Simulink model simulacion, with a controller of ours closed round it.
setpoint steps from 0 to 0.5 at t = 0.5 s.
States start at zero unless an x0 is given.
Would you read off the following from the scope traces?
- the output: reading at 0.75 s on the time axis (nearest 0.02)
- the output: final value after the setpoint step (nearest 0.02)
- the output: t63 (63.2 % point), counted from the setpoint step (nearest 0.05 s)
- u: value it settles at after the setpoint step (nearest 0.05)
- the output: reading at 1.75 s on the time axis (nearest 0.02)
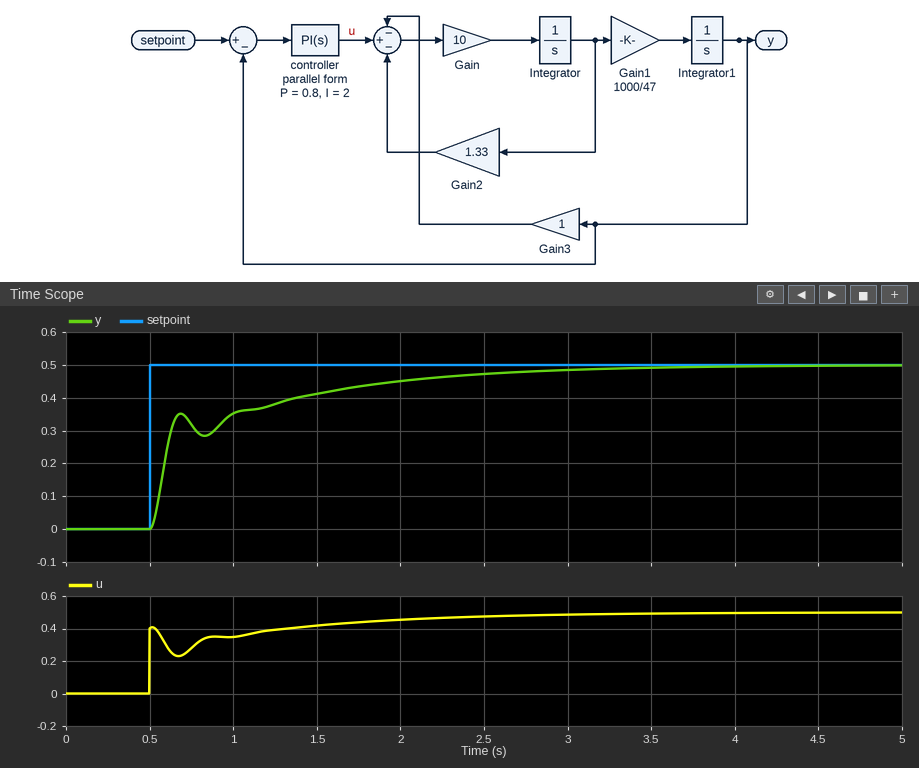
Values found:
0.32
0.50
0.15 s
0.50
0.44
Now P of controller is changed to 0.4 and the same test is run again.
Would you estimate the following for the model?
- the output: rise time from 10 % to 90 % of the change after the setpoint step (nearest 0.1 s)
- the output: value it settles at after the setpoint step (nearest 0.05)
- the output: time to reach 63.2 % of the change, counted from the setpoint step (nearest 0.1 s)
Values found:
1.3 s
0.50
0.5 s
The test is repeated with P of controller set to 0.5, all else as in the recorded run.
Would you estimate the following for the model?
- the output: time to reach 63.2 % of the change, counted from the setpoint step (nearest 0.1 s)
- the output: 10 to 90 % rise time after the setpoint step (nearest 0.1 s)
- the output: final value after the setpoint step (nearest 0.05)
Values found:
0.5 s
1.3 s
0.50
